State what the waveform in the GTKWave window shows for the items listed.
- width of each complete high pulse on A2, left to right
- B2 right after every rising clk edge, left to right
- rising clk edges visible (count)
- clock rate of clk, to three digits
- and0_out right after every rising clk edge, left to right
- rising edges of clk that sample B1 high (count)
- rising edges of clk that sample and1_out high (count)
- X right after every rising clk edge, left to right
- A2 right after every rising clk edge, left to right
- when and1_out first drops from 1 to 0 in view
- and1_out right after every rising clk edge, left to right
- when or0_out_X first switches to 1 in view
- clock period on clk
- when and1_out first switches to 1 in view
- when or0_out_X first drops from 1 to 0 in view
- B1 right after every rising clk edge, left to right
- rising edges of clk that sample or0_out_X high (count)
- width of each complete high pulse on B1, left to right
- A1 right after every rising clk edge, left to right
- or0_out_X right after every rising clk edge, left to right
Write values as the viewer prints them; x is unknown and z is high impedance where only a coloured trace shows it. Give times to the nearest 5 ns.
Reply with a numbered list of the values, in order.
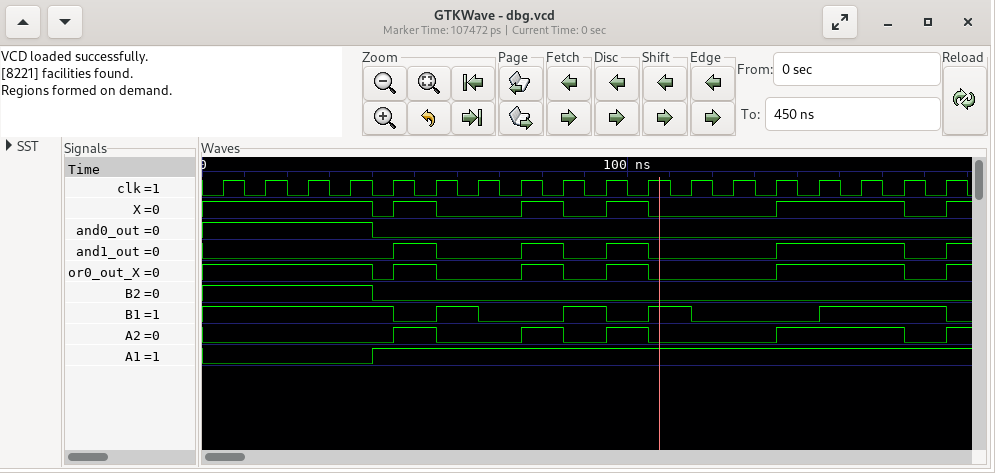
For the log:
1. 10 ns, 10 ns, 10 ns, 30 ns
2. 1 1 1 1 0 0 0 0 0 0 0 0 0 0 0 0 0 0
3. 18
4. 100 MHz
5. 1 1 1 1 0 0 0 0 0 0 0 0 0 0 0 0 0 0
6. 11
7. 6
8. 1 1 1 1 1 0 0 1 0 1 0 0 0 1 1 1 0 1
9. 0 0 0 0 1 0 0 1 0 1 0 0 0 1 1 1 0 1
10. 55 ns
11. 0 0 0 0 1 0 0 1 0 1 0 0 0 1 1 1 0 1
12. 45 ns
13. 10 ns
14. 45 ns
15. 40 ns
16. 1 1 1 1 0 1 0 0 1 0 1 0 0 0 1 1 1 0
17. 10
18. 10 ns, 10 ns, 10 ns, 30 ns
19. 0 0 0 0 1 1 1 1 1 1 1 1 1 1 1 1 1 1
20. 1 1 1 1 1 0 0 1 0 1 0 0 0 1 1 1 0 1
